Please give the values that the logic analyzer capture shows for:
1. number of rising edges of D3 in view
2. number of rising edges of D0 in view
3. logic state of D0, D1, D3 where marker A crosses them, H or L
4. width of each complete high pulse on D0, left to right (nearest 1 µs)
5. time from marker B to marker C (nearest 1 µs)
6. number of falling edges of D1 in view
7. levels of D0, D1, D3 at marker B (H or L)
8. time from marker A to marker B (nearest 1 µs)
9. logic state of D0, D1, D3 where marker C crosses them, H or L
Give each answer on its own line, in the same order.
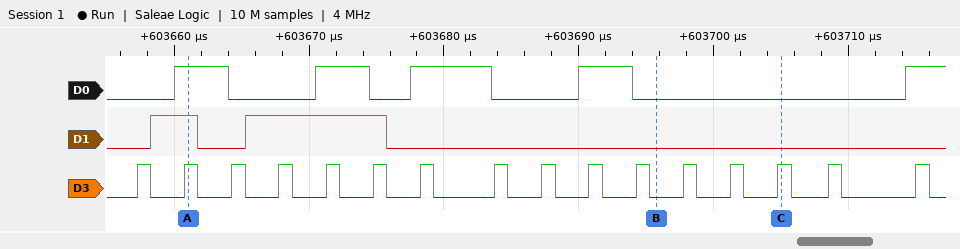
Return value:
16
5
D0=H, D1=H, D3=H
4 µs, 4 µs, 6 µs, 4 µs
9 µs
2
D0=L, D1=L, D3=L
35 µs
D0=L, D1=L, D3=H
